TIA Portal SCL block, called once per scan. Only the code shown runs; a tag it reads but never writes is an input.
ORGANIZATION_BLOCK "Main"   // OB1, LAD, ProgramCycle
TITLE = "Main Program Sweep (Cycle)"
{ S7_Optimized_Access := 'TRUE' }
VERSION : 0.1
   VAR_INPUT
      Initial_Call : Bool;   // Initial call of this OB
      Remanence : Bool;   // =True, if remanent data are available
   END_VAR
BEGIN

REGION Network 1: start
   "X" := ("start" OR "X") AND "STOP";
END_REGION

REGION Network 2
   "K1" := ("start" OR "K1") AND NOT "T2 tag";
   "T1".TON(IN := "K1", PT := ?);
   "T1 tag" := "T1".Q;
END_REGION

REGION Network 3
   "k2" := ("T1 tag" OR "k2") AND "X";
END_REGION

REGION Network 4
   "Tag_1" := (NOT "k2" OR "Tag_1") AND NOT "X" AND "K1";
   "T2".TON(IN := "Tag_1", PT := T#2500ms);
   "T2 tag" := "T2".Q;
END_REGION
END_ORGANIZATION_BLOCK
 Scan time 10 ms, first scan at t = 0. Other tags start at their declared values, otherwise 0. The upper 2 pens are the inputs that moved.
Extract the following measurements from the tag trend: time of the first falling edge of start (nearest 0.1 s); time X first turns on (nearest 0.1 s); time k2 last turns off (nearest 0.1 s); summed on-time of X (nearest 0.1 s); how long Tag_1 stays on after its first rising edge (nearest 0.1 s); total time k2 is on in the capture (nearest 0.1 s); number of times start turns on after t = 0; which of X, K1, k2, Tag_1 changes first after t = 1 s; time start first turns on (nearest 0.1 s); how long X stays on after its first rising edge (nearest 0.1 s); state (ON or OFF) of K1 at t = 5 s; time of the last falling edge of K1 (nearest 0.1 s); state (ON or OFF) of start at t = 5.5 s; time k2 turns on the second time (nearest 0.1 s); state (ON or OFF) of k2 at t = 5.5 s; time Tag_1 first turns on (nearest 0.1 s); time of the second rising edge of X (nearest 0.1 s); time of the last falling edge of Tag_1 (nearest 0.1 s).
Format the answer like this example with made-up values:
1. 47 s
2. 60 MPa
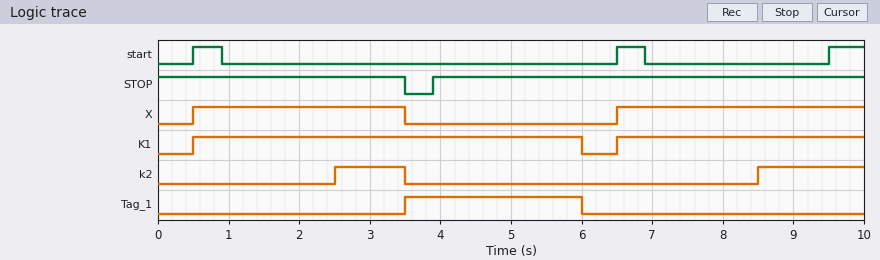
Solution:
1. 0.9 s
2. 0.5 s
3. 3.5 s
4. 6.5 s
5. 2.5 s
6. 2.5 s
7. 3
8. k2
9. 0.5 s
10. 3.0 s
11. ON
12. 6.0 s
13. OFF
14. 8.5 s
15. OFF
16. 3.5 s
17. 6.5 s
18. 6.0 s
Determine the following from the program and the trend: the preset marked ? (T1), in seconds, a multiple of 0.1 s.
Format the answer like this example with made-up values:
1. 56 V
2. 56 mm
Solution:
1. 2.0 s
